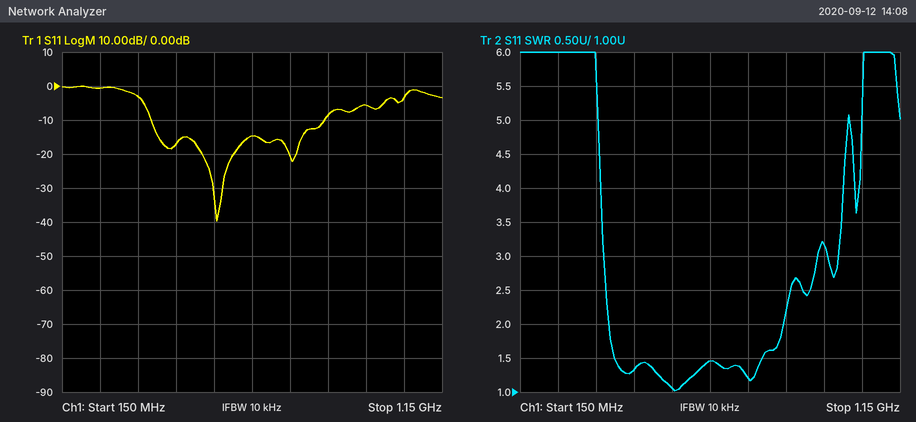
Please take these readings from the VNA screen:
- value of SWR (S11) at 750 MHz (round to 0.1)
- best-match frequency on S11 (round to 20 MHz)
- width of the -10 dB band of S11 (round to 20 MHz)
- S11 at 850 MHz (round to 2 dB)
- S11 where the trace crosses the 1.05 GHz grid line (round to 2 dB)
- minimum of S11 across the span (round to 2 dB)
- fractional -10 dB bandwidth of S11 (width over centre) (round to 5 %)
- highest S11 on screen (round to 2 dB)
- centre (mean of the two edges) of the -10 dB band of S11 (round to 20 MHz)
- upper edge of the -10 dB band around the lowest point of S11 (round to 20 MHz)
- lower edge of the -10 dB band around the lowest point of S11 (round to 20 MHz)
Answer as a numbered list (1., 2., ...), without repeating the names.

1. 1.2
2. 560 MHz
3. 460 MHz
4. -8 dB
5. -4 dB
6. -40 dB
7. 75 %
8. 0 dB
9. 620 MHz
10. 840 MHz
11. 380 MHz
